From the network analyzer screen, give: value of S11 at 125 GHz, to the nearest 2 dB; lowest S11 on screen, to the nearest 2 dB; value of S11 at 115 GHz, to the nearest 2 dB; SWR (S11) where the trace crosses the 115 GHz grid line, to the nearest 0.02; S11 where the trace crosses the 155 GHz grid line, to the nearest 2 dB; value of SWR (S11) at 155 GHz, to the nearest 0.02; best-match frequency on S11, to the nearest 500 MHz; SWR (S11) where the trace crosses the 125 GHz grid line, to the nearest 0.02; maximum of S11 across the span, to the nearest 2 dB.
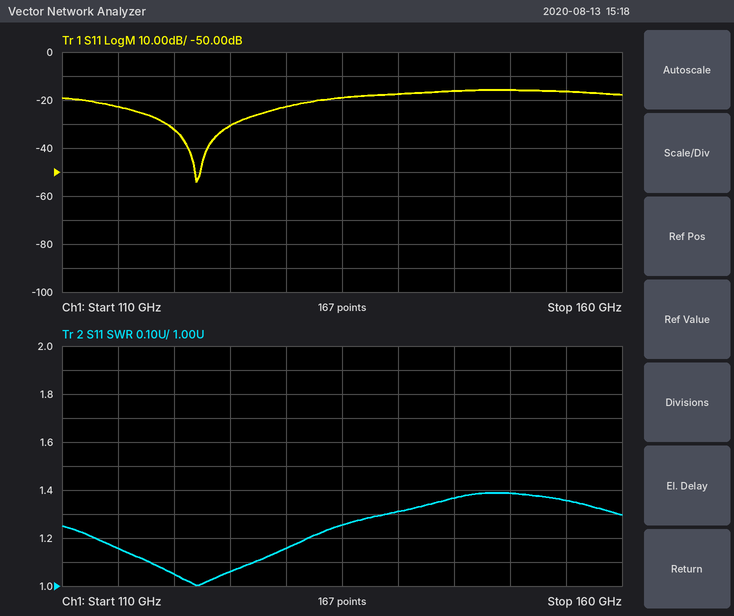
-30 dB
-54 dB
-22 dB
1.16
-16 dB
1.36
122.0 GHz
1.06
-16 dB
